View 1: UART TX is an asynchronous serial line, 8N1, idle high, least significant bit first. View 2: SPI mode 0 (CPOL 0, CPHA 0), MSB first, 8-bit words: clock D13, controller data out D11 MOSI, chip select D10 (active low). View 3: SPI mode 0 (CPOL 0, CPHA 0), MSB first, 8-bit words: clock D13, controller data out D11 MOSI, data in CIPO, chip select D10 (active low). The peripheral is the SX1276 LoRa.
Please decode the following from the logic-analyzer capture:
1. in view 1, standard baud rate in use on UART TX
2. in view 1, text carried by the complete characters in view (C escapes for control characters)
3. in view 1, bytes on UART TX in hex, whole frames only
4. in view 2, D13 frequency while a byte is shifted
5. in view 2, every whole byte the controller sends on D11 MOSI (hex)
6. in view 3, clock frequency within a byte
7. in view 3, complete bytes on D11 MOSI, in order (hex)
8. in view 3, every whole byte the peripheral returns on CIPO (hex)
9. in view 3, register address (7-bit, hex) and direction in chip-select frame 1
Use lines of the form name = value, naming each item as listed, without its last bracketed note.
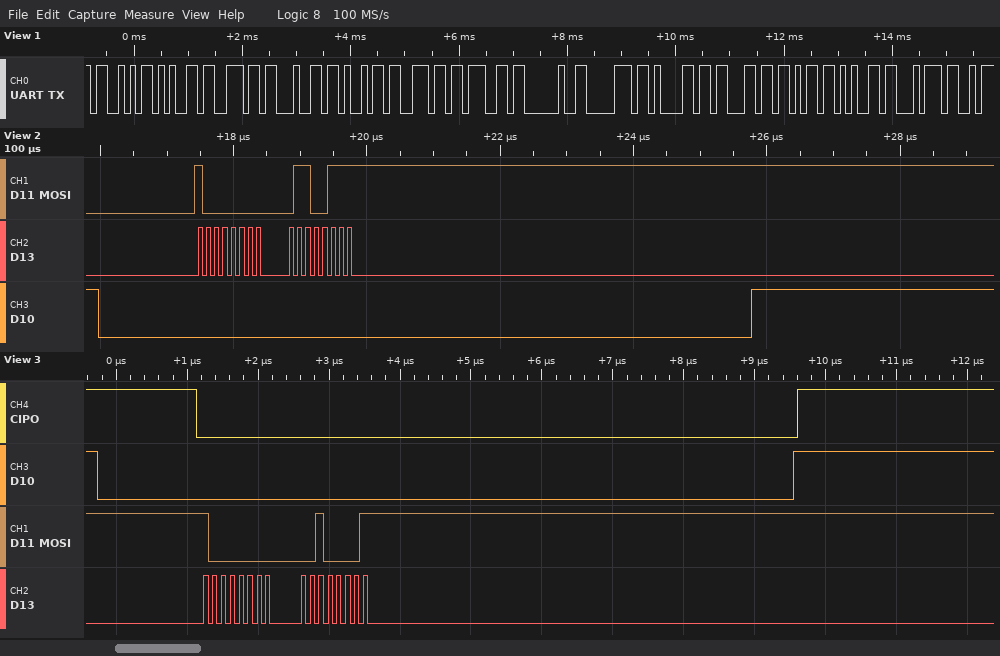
in view 1, standard baud rate in use on UART TX = 9600 baud
in view 1, text carried by the complete characters in view = "Sending packet"
in view 1, bytes on UART TX in hex, whole frames only = 53 65 6E 64 69 6E 67 20 70 61 63 6B 65 74
in view 2, D13 frequency while a byte is shifted = 8 MHz
in view 2, every whole byte the controller sends on D11 MOSI = 0x80 0x67
in view 3, clock frequency within a byte = 8 MHz
in view 3, complete bytes on D11 MOSI, in order = 0x80 0x21
in view 3, every whole byte the peripheral returns on CIPO = 0x00 0x00
in view 3, register address (7-bit, hex) and direction in chip-select frame 1 = 0x00 write
